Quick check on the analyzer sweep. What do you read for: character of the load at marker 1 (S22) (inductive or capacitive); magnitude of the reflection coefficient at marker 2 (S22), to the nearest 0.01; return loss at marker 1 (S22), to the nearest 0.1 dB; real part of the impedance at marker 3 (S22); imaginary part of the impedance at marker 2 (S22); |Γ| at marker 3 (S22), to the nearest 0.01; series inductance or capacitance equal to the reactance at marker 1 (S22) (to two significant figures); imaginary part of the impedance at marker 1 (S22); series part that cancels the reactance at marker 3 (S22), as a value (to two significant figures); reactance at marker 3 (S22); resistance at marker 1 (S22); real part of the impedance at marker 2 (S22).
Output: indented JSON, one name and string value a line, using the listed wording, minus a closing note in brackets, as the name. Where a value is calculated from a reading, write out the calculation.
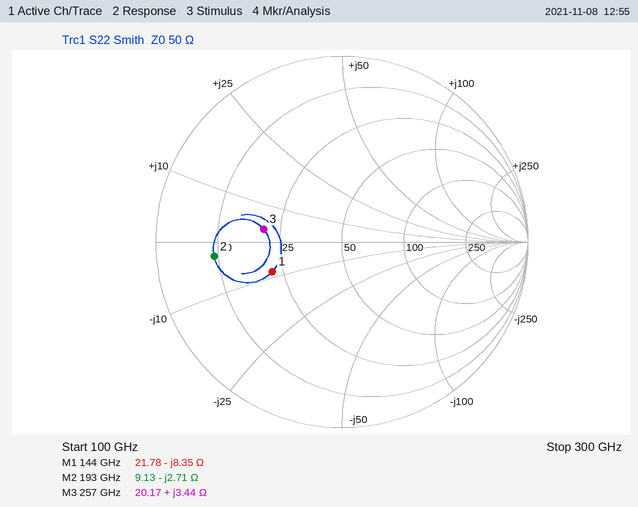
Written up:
{
  "character of the load at marker 1 (S22)": "capacitive",
  "magnitude of the reflection coefficient at marker 2 (S22), to the nearest 0.01": "0.69",
  "return loss at marker 1 (S22), to the nearest 0.1 dB": "7.8 dB",
  "real part of the impedance at marker 3": "20.17 Ω",
  "imaginary part of the impedance at marker 2": "-2.71 Ω",
  "|Γ| at marker 3 (S22), to the nearest 0.01": "0.43",
  "series inductance or capacitance equal to the reactance at marker 1 (S22)": "C = 1/(2π × 144 GHz × 8.35 Ω) ≈ 132 fF, so 130 fF to two significant figures",
  "imaginary part of the impedance at marker 1": "-8.35 Ω",
  "series part that cancels the reactance at marker 3 (S22), as a value": "C = 1/(2π × 257 GHz × 3.44 Ω) ≈ 180 fF",
  "reactance at marker 3": "+3.44 Ω",
  "resistance at marker 1": "21.78 Ω",
  "real part of the impedance at marker 2": "9.13 Ω"
}
